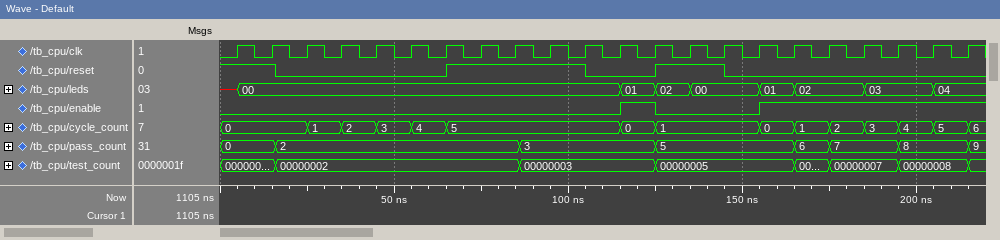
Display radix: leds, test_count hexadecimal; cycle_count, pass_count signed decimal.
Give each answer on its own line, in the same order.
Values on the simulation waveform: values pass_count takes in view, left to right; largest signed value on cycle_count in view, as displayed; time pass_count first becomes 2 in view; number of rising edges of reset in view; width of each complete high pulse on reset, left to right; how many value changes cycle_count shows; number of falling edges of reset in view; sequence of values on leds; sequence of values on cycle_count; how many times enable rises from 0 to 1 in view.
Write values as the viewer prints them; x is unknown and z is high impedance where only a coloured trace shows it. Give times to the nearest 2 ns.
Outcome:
0, 2, 3, 5, 6, 7, 8, 9
6
16 ns
2
40 ns, 20 ns
14
3
x, 00, 01, 02, 00, 01, 02, 03, 04
0, 1, 2, 3, 4, 5, 0, 1, 0, 1, 2, 3, 4, 5, 6
2
